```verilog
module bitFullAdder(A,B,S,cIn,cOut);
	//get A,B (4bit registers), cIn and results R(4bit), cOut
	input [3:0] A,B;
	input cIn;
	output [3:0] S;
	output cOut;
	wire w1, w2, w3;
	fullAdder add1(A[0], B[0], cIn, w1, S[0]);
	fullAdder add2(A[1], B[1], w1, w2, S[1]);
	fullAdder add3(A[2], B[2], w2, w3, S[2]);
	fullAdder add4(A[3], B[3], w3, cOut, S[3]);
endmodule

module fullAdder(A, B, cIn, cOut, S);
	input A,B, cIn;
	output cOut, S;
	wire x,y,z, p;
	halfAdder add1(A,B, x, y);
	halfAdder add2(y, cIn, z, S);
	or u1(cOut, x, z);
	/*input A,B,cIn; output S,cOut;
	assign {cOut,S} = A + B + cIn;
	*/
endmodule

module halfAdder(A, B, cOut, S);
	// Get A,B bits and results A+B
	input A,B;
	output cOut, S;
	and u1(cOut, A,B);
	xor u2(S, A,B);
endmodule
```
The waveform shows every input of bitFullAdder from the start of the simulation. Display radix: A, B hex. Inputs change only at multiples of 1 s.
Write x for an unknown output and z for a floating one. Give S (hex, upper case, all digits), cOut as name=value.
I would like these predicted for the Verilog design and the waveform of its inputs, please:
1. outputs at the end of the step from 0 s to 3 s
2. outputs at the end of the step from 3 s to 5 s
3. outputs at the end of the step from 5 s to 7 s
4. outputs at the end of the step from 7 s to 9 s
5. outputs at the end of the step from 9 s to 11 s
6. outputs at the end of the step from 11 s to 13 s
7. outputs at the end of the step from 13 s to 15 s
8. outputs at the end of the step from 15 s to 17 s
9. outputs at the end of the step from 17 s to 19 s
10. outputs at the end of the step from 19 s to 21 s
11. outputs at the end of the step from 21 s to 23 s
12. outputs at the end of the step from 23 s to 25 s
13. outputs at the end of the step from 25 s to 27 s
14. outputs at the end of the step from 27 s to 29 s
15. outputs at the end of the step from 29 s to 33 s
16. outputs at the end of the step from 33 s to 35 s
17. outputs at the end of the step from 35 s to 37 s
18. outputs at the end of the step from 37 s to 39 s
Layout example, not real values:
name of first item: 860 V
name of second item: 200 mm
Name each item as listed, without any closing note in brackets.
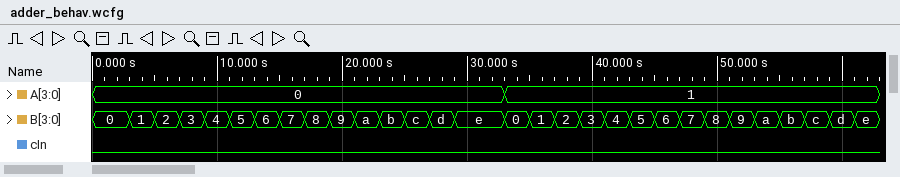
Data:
outputs at the end of the step from 0 s to 3 s: S=0, cOut=0
outputs at the end of the step from 3 s to 5 s: S=1, cOut=0
outputs at the end of the step from 5 s to 7 s: S=2, cOut=0
outputs at the end of the step from 7 s to 9 s: S=3, cOut=0
outputs at the end of the step from 9 s to 11 s: S=4, cOut=0
outputs at the end of the step from 11 s to 13 s: S=5, cOut=0
outputs at the end of the step from 13 s to 15 s: S=6, cOut=0
outputs at the end of the step from 15 s to 17 s: S=7, cOut=0
outputs at the end of the step from 17 s to 19 s: S=8, cOut=0
outputs at the end of the step from 19 s to 21 s: S=9, cOut=0
outputs at the end of the step from 21 s to 23 s: S=A, cOut=0
outputs at the end of the step from 23 s to 25 s: S=B, cOut=0
outputs at the end of the step from 25 s to 27 s: S=C, cOut=0
outputs at the end of the step from 27 s to 29 s: S=D, cOut=0
outputs at the end of the step from 29 s to 33 s: S=E, cOut=0
outputs at the end of the step from 33 s to 35 s: S=1, cOut=0
outputs at the end of the step from 35 s to 37 s: S=2, cOut=0
outputs at the end of the step from 37 s to 39 s: S=3, cOut=0
